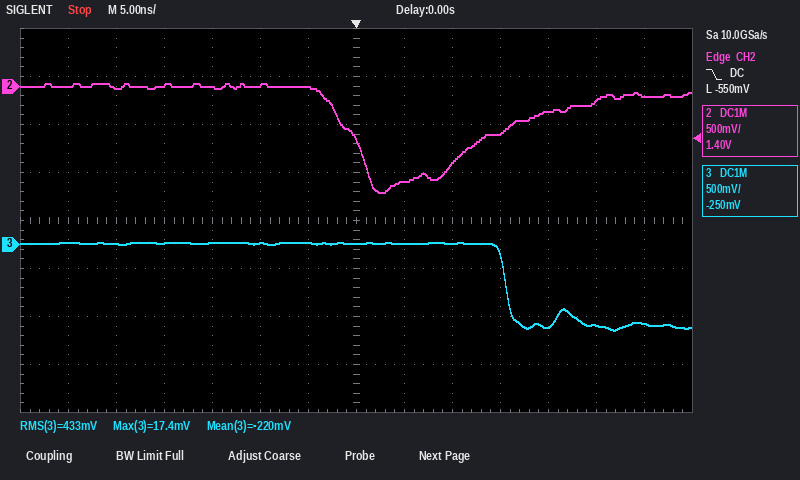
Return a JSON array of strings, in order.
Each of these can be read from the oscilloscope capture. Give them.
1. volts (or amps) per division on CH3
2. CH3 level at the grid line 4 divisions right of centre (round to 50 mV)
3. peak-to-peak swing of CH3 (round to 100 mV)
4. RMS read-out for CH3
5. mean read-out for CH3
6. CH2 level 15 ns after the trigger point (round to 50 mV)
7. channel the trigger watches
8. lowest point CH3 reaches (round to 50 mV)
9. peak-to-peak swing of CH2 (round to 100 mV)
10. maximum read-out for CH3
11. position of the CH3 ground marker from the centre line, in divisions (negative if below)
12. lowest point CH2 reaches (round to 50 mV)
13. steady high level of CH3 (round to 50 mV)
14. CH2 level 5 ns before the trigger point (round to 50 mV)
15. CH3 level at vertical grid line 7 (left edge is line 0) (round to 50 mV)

["500 mV", "-850 mV", "900 mV", "433 mV", "-220 mV", "-500 mV", "CH2", "-900 mV", "1.10 V", "17.4 mV", "-0.5 div", "-1.10 V", "0 mV", "0 mV", "0 mV"]
